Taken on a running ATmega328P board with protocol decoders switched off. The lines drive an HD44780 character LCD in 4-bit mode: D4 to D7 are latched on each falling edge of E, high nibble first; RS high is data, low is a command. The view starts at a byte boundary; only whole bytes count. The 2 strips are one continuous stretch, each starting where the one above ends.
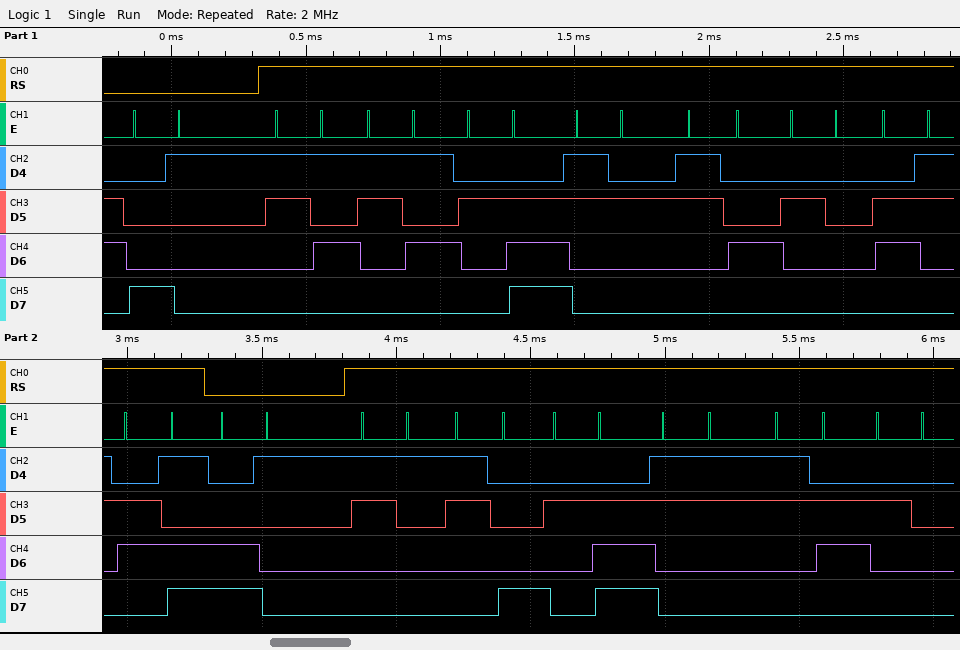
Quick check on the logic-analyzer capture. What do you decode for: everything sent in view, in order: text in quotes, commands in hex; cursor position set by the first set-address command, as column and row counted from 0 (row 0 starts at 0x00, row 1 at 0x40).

0x81 "55.24 cm" 0xC1 "18.36 "
column 1, row 0
